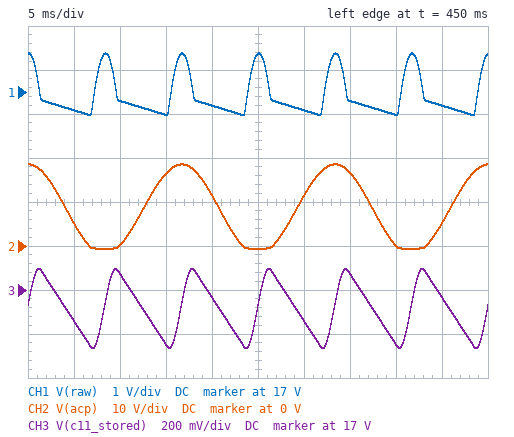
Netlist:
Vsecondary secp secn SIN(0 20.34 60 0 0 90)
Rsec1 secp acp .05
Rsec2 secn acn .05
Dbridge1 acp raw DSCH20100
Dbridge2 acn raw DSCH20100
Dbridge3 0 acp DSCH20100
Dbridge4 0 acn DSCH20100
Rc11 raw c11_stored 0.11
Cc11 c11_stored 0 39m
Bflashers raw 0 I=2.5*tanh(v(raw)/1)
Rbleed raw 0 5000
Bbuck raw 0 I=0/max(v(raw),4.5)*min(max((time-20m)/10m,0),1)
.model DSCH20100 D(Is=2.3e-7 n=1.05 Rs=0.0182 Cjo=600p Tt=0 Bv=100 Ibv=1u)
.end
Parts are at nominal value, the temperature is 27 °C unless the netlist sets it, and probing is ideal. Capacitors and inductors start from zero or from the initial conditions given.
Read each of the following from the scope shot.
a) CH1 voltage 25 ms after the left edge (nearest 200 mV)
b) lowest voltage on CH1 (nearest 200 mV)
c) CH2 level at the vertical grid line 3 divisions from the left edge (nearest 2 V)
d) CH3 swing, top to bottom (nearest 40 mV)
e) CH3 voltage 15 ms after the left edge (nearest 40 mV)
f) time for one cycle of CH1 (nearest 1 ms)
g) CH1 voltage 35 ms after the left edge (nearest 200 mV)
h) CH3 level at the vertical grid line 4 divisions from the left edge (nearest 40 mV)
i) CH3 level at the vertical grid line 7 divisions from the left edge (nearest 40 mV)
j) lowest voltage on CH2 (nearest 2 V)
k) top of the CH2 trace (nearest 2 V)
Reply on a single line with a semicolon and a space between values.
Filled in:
17.8 V; 16.4 V; 16 V; 360 mV; 16.76 V; 8 ms; 16.8 V; 16.96 V; 17.08 V; 0 V; 18 V
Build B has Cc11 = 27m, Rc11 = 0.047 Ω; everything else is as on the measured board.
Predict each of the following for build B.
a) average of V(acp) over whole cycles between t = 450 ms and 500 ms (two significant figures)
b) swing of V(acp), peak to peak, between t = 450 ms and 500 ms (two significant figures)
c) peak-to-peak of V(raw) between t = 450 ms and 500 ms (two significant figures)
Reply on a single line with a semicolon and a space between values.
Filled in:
8.6 V; 19 V; 910 mV
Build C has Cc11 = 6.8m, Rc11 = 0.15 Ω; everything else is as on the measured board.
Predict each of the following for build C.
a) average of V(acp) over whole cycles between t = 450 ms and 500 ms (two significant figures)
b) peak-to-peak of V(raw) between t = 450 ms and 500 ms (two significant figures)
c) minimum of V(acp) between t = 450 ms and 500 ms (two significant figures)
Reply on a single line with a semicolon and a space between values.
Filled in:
8.3 V; 2.9 V; -670 mV
